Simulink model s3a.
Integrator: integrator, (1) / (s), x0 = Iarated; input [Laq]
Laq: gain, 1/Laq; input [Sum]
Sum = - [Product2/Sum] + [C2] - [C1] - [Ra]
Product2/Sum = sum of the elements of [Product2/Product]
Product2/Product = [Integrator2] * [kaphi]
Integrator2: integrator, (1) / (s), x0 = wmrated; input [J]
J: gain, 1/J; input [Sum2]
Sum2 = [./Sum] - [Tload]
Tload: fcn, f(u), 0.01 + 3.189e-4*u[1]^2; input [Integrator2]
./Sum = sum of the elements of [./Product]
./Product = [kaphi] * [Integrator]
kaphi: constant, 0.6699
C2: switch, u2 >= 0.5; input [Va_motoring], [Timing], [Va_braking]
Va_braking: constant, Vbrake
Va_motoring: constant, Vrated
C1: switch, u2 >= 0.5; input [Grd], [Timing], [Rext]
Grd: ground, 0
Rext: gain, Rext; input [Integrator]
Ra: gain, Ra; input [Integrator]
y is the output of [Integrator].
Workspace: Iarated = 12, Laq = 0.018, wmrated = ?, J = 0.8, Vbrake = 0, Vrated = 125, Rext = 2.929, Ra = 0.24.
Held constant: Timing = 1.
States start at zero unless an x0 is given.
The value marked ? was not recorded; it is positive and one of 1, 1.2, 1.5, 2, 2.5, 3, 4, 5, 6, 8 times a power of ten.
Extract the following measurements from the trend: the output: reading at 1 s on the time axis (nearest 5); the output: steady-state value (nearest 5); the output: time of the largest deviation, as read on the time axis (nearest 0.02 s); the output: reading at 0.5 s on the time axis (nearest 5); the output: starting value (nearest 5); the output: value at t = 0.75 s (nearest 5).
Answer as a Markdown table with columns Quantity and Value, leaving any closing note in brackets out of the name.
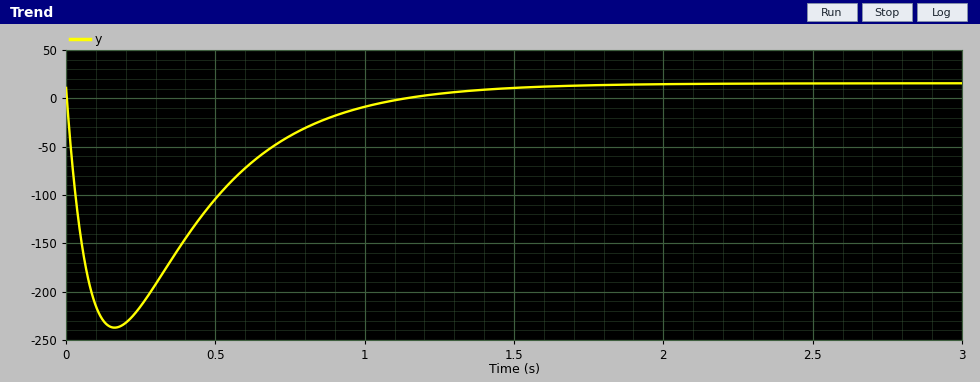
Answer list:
| Quantity | Value |
|---|---|
| the output: reading at 1 s on the time axis | -10 |
| the output: steady-state value | 15 |
| the output: time of the largest deviation, as read on the time axis | 0.16 s |
| the output: reading at 0.5 s on the time axis | -105 |
| the output: starting value | 10 |
| the output: value at t = 0.75 s | -40 |
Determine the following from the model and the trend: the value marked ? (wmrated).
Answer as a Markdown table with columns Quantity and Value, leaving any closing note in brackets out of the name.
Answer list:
| Quantity | Value |
|---|---|
| the value marked ? | 300 |
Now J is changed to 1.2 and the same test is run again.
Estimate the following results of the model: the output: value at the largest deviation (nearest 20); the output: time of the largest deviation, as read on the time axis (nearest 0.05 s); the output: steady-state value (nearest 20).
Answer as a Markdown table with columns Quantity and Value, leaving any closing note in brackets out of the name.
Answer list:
| Quantity | Value |
|---|---|
| the output: value at the largest deviation | -260 |
| the output: time of the largest deviation, as read on the time axis | 0.20 s |
| the output: steady-state value | 20 |
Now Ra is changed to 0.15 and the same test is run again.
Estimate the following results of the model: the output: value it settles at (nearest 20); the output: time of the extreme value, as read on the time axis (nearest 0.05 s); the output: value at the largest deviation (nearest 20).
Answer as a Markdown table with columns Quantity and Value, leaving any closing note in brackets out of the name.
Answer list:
| Quantity | Value |
|---|---|
| the output: value it settles at | 20 |
| the output: time of the extreme value, as read on the time axis | 0.20 s |
| the output: value at the largest deviation | -320 |
